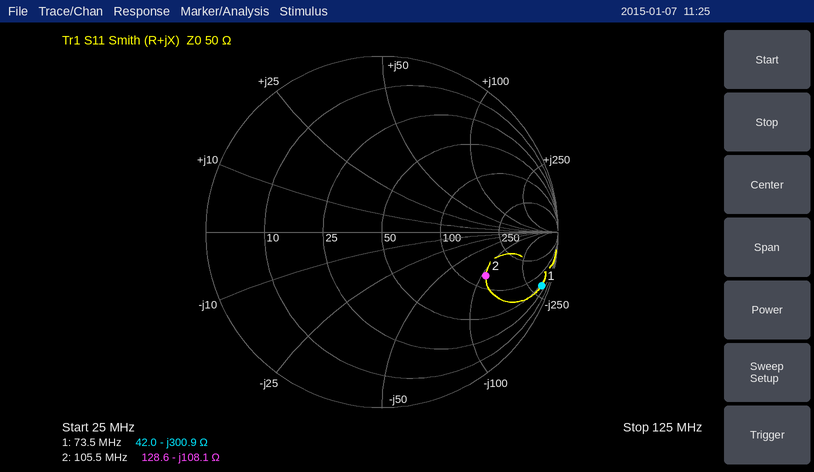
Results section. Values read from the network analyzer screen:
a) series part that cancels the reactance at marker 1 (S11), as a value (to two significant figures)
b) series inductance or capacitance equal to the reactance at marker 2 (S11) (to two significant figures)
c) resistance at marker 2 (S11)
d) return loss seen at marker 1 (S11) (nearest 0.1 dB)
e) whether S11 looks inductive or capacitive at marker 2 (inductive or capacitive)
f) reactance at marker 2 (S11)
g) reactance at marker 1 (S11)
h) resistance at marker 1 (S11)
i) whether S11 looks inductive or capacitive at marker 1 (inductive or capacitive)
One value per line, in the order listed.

650 nH
14 pF
128.6 Ω
0.4 dB
capacitive
-108.1 Ω
-300.9 Ω
42.0 Ω
capacitive
